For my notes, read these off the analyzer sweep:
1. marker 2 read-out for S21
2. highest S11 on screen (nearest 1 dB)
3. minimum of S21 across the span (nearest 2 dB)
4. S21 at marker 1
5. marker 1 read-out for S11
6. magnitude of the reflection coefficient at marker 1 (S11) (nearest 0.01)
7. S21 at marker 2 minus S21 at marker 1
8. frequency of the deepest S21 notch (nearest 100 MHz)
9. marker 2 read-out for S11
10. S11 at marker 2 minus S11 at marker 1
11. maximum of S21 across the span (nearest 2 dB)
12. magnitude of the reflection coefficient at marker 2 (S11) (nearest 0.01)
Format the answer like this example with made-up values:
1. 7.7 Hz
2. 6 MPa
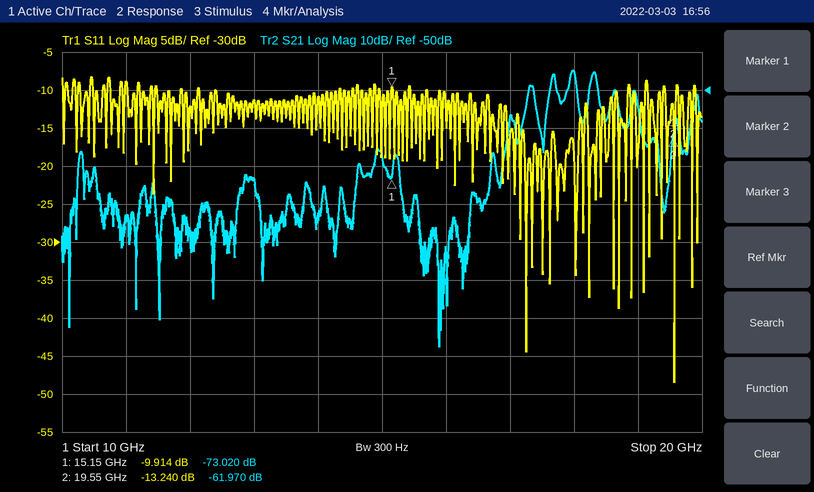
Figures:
1. -61.970 dB
2. -8 dB
3. -118 dB
4. -73.020 dB
5. -9.914 dB
6. 0.32
7. 11.050 dB
8. 15.9 GHz
9. -13.240 dB
10. -3.326 dB
11. -44 dB
12. 0.22
